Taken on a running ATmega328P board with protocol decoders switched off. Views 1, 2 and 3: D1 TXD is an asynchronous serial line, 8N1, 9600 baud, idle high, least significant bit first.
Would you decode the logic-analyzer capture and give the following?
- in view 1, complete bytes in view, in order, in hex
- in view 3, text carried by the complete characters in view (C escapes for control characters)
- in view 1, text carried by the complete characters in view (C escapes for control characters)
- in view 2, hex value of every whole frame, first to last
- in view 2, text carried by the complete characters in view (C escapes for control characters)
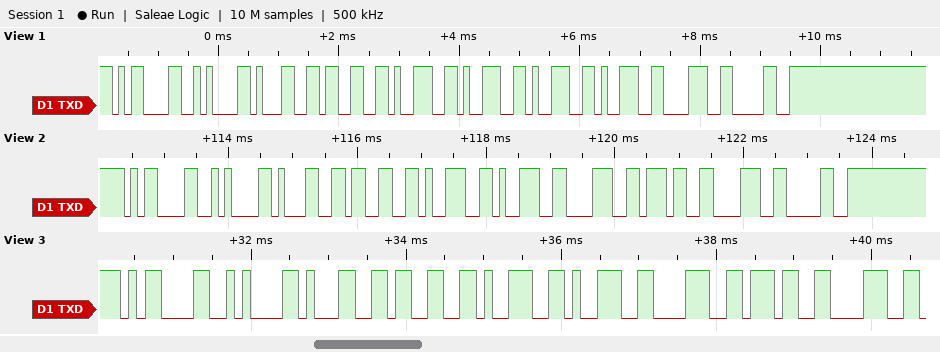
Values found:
0D 0A 31 33 39 39 39 39 38 30
"\r\n1399878"
"\r\n13999980"
0x0D 0x0A 0x31 0x33 0x39 0x39 0x38 0x37 0x38 0x30
"\r\n13998780"
